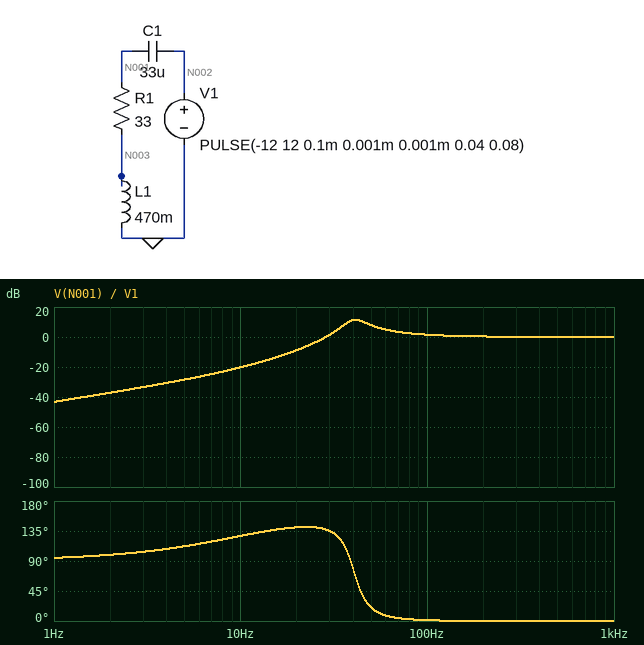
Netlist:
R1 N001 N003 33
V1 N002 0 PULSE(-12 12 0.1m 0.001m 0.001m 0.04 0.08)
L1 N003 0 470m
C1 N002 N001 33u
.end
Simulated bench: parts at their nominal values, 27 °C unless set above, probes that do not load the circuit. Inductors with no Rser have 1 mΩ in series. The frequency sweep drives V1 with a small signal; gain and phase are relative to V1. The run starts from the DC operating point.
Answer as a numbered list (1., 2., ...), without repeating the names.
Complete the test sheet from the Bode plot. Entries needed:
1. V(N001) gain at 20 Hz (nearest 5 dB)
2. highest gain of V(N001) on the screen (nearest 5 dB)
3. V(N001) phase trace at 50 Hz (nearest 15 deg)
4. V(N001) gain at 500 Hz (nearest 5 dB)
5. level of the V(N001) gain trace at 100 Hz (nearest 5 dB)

1. -10 dB
2. 10 dB
3. 15 deg
4. 0 dB
5. 0 dB
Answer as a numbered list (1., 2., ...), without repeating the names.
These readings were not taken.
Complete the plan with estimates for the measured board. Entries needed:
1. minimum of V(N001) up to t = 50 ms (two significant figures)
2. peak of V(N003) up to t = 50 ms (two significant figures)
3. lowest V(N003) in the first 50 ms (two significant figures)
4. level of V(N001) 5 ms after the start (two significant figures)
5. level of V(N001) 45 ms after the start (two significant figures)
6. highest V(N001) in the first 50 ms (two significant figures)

1. -29 V
2. 24 V
3. -28 V
4. 9.4 V
5. -8.6 V
6. 24 V
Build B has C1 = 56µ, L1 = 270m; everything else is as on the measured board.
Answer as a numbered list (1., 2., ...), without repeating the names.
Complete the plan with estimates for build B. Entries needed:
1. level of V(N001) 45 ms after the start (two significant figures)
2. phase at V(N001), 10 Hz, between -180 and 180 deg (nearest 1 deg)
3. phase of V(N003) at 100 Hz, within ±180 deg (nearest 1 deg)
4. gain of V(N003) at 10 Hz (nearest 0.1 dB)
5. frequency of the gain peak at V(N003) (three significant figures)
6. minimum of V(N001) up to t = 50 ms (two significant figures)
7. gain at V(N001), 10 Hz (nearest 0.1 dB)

1. -10 V
2. 110 deg
3. 13 deg
4. -24.0 dB
5. 43.5 Hz
6. -26 V
7. -17.2 dB
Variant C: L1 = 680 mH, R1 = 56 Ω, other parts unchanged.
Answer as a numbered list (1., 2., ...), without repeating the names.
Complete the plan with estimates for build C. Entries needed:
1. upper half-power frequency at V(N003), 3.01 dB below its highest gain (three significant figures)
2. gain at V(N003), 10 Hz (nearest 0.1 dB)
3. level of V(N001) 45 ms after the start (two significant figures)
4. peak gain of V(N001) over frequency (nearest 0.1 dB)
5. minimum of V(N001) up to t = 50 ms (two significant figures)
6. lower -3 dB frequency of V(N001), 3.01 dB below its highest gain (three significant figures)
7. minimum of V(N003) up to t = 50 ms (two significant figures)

1. 45.7 Hz
2. -20.3 dB
3. -17 V
4. 8.9 dB
5. -25 V
6. 29.2 Hz
7. -27 V
